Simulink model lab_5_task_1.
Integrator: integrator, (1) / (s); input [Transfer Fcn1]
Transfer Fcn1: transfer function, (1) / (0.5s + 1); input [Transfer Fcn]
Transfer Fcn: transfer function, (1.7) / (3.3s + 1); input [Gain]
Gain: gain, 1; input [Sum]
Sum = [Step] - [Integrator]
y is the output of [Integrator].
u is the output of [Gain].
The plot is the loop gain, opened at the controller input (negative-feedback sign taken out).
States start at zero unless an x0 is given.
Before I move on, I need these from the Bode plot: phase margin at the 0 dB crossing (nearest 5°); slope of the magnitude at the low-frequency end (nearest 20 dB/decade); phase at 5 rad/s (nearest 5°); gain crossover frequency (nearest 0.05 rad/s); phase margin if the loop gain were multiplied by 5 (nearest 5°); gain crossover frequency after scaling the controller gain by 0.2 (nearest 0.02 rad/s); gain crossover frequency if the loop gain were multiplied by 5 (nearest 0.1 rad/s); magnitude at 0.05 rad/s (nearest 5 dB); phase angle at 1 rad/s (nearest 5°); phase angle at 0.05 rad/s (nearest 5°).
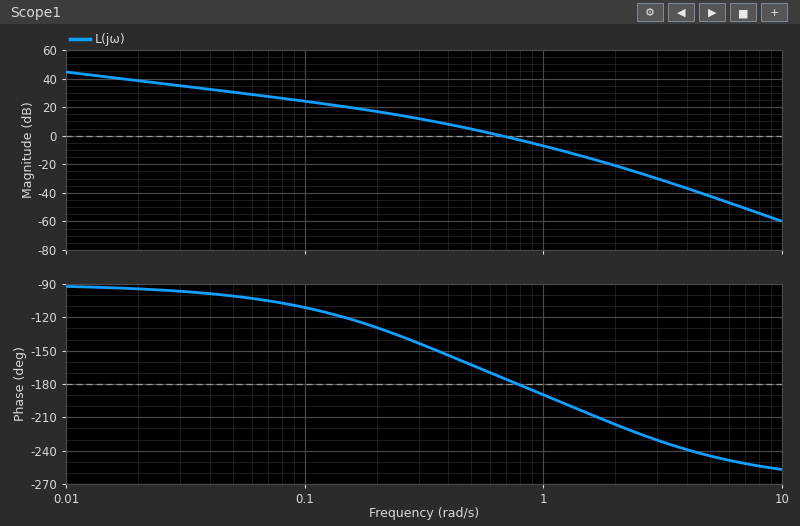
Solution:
5°
-20 dB/decade
-245°
0.65 rad/s
-25°
0.26 rad/s
1.4 rad/s
30 dB
-190°
-100°
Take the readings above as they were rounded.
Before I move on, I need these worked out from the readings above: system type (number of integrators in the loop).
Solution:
1
